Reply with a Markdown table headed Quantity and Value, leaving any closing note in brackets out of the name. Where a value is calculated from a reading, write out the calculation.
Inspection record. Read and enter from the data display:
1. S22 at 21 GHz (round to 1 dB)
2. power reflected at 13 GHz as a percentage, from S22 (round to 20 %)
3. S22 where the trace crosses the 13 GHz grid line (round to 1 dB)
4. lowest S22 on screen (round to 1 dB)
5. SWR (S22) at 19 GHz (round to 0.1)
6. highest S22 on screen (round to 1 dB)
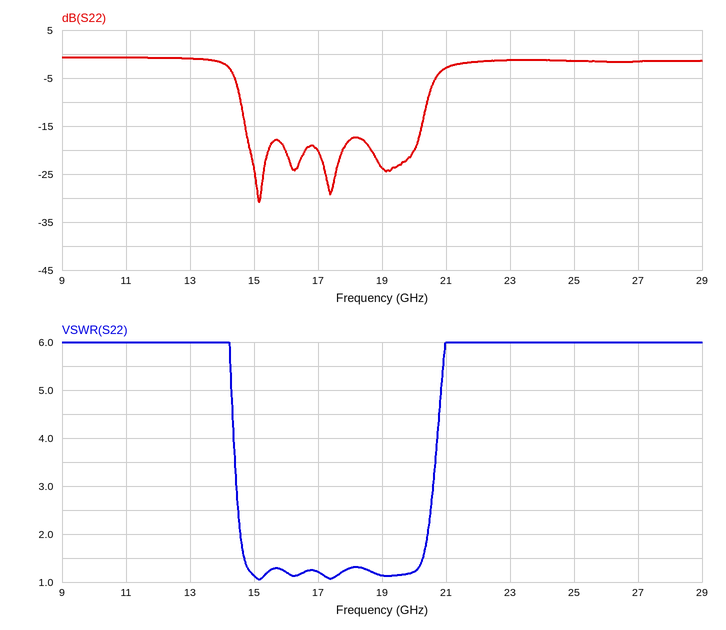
| Quantity | Value |
|---|---|
| S22 at 21 GHz | -3 dB |
| power reflected at 13 GHz as a percentage, from S22 | 10^(-1/10) ≈ 79.4 %, so 80 % to the nearest 20 % |
| S22 where the trace crosses the 13 GHz grid line | -1 dB |
| lowest S22 on screen | -31 dB |
| SWR (S22) at 19 GHz | 1.1 |
| highest S22 on screen | -1 dB |
